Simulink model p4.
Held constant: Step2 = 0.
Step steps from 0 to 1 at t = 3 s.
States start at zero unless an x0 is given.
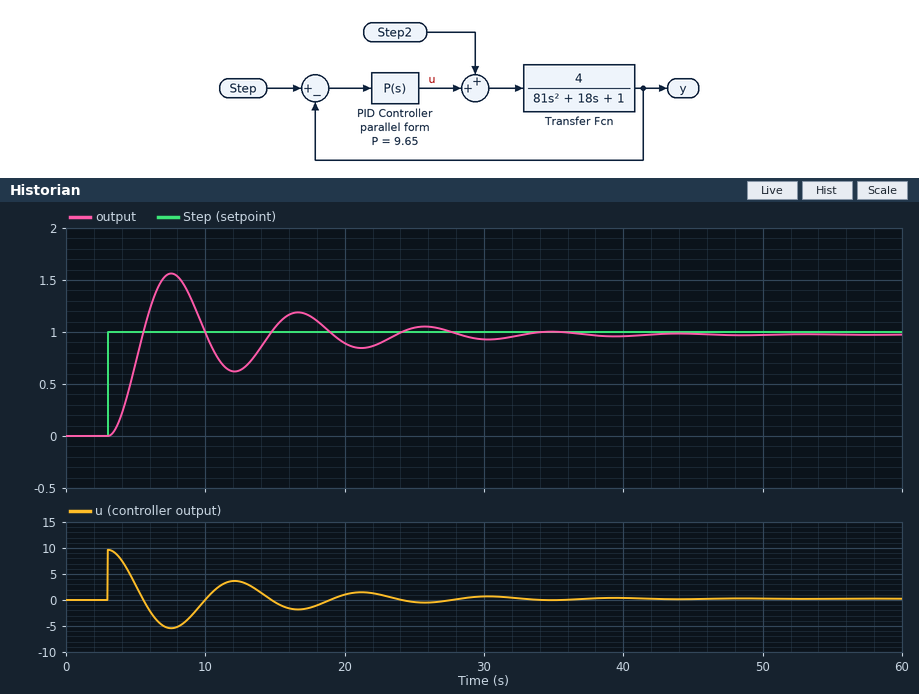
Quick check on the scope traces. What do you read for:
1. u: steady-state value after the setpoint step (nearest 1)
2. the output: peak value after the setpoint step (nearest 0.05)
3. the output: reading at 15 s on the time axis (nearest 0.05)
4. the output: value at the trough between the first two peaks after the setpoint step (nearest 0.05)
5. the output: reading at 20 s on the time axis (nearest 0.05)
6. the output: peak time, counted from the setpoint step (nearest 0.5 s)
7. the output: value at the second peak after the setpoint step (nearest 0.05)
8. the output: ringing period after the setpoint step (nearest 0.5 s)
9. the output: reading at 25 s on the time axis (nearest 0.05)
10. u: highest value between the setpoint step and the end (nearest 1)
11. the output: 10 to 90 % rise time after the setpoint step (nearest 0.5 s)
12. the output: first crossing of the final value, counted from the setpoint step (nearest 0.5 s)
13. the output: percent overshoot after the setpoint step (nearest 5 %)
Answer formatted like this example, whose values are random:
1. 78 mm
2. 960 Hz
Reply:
1. 0
2. 1.55
3. 1.05
4. 0.60
5. 0.90
6. 4.5 s
7. 1.20
8. 9.0 s
9. 1.05
10. 10
11. 1.5 s
12. 2.5 s
13. 60 %
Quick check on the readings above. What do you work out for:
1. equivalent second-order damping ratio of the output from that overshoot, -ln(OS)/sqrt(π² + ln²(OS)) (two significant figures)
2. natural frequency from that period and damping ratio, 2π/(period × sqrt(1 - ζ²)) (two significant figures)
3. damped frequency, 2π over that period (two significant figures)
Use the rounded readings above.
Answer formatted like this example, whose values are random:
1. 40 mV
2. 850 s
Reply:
1. 0.16
2. 0.71 rad/s
3. 0.70 rad/s
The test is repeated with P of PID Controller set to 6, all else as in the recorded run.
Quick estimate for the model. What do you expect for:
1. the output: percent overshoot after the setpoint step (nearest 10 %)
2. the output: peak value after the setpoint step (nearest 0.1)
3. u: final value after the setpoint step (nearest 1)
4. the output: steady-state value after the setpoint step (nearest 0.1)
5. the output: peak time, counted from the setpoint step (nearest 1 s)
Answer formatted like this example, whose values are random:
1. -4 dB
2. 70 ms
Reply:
1. 50 %
2. 1.5
3. 0
4. 1.0
5. 6 s
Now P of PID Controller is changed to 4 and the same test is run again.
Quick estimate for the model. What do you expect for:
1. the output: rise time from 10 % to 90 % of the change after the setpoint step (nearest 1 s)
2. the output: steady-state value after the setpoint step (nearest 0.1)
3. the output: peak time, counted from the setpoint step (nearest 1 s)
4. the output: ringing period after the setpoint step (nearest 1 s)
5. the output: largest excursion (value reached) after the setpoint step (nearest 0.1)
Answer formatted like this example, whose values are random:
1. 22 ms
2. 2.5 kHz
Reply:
1. 3 s
2. 0.9
3. 7 s
4. 14 s
5. 1.4
